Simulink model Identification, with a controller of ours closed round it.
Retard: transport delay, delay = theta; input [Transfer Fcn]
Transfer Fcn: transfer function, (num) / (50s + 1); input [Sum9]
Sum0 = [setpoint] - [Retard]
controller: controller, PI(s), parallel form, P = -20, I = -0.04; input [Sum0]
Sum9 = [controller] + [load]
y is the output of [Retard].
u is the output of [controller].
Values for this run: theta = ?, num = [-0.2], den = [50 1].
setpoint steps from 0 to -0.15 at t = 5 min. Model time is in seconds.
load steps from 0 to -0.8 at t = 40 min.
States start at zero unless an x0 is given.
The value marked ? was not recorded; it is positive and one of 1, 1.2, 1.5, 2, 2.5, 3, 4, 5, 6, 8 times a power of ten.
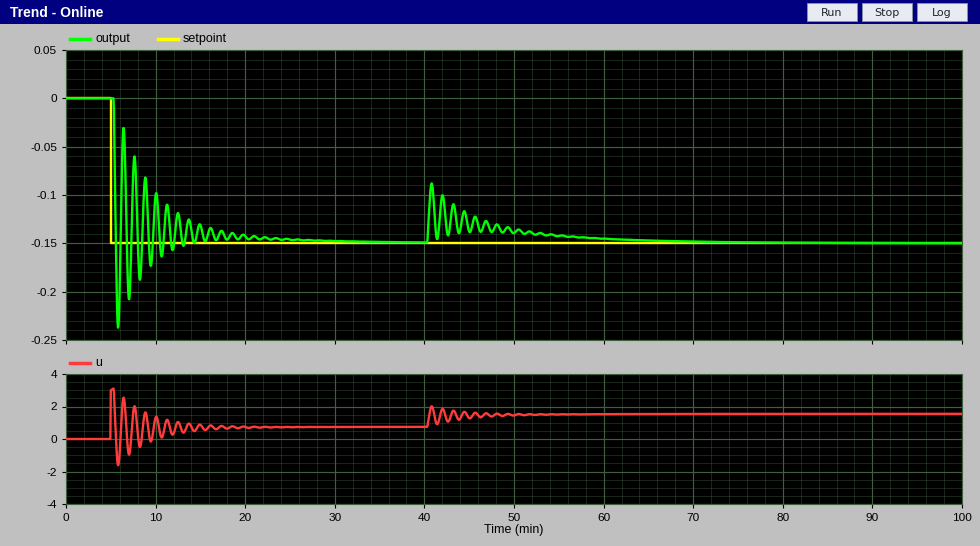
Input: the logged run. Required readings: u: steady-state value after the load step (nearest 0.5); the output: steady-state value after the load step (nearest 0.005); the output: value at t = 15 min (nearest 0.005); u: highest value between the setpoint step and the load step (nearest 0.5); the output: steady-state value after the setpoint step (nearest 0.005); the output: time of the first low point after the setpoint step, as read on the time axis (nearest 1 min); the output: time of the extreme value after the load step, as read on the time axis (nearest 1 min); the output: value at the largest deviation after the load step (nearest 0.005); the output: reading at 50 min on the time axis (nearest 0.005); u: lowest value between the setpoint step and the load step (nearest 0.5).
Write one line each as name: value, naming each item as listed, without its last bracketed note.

u: steady-state value after the load step: 1.5
the output: steady-state value after the load step: -0.150
the output: value at t = 15 min: -0.130
u: highest value between the setpoint step and the load step: 3.0
the output: steady-state value after the setpoint step: -0.150
the output: time of the first low point after the setpoint step, as read on the time axis: 6 min
the output: time of the extreme value after the load step, as read on the time axis: 41 min
the output: value at the largest deviation after the load step: -0.090
the output: reading at 50 min on the time axis: -0.140
u: lowest value between the setpoint step and the load step: -1.5
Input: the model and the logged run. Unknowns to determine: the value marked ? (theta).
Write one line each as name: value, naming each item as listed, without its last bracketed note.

the value marked ?: 20
